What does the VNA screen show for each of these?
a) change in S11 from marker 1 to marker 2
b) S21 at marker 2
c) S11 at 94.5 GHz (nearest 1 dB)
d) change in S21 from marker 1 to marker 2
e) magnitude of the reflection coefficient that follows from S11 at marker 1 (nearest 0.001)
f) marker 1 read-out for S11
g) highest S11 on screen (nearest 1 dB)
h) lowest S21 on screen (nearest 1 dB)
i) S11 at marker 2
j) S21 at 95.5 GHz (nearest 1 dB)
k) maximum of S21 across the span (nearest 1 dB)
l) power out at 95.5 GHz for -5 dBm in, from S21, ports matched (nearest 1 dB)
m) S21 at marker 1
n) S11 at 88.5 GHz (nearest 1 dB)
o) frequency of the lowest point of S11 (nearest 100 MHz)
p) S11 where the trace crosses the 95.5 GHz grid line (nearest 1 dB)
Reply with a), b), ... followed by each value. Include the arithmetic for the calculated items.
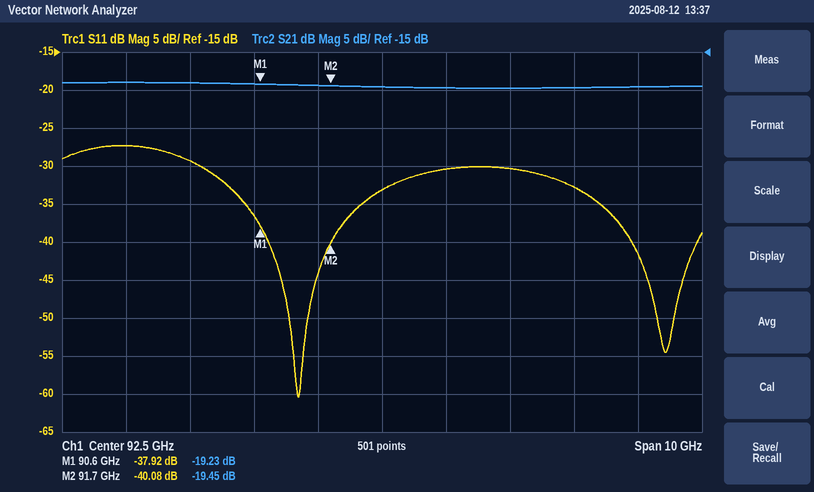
a) -40.08 − (-37.92) = -2.16 dB
b) -19.45 dB
c) -30 dB
d) -19.45 − (-19.23) = -0.22 dB
e) 10^(-37.92/20) ≈ 0.013
f) -37.92 dB
g) -27 dB
h) -20 dB
i) -40.08 dB
j) -20 dB
k) -19 dB
l) -5 dBm + (-20 dB) = -25 dBm
m) -19.23 dB
n) -27 dB
o) 91.2 GHz
p) -33 dB
